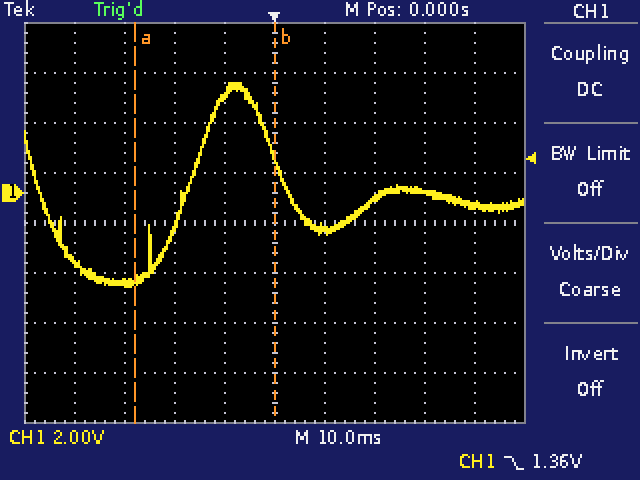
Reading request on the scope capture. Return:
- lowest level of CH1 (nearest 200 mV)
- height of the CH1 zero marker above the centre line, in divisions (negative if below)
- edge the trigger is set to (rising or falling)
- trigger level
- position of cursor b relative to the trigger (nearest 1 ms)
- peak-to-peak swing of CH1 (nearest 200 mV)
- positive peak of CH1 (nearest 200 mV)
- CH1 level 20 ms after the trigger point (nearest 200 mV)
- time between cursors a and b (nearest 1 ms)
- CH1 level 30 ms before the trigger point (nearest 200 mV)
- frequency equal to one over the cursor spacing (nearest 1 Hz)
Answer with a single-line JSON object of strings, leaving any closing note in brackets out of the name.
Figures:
{"lowest level of CH1": "-3.8 V", "height of the CH1 zero marker above the centre line, in divisions": "+0.6 div", "edge the trigger is set to": "falling", "trigger level": "1.36 V", "position of cursor b relative to the trigger": "0 ms", "peak-to-peak swing of CH1": "8.2 V", "positive peak of CH1": "4.4 V", "CH1 level 20 ms after the trigger point": "-200 mV", "time between cursors a and b": "28 ms", "CH1 level 30 ms before the trigger point": "-3.6 V", "frequency equal to one over the cursor spacing": "36 Hz"}
